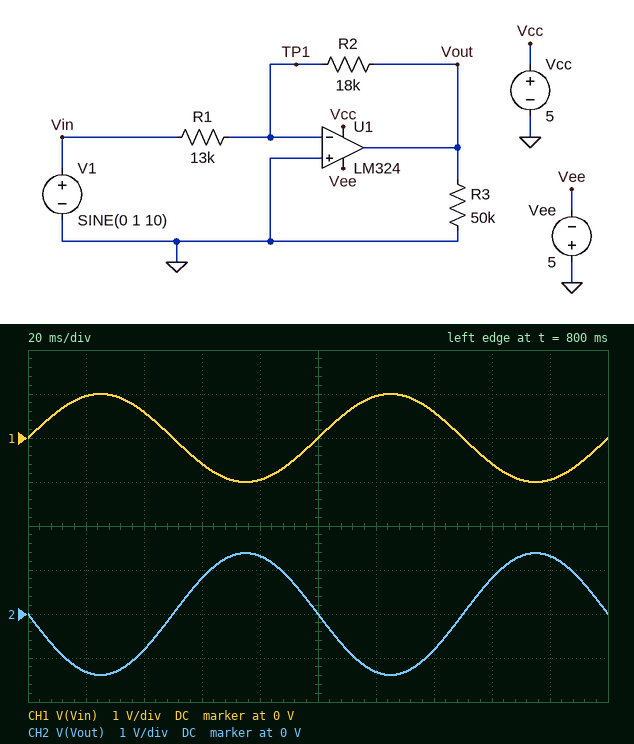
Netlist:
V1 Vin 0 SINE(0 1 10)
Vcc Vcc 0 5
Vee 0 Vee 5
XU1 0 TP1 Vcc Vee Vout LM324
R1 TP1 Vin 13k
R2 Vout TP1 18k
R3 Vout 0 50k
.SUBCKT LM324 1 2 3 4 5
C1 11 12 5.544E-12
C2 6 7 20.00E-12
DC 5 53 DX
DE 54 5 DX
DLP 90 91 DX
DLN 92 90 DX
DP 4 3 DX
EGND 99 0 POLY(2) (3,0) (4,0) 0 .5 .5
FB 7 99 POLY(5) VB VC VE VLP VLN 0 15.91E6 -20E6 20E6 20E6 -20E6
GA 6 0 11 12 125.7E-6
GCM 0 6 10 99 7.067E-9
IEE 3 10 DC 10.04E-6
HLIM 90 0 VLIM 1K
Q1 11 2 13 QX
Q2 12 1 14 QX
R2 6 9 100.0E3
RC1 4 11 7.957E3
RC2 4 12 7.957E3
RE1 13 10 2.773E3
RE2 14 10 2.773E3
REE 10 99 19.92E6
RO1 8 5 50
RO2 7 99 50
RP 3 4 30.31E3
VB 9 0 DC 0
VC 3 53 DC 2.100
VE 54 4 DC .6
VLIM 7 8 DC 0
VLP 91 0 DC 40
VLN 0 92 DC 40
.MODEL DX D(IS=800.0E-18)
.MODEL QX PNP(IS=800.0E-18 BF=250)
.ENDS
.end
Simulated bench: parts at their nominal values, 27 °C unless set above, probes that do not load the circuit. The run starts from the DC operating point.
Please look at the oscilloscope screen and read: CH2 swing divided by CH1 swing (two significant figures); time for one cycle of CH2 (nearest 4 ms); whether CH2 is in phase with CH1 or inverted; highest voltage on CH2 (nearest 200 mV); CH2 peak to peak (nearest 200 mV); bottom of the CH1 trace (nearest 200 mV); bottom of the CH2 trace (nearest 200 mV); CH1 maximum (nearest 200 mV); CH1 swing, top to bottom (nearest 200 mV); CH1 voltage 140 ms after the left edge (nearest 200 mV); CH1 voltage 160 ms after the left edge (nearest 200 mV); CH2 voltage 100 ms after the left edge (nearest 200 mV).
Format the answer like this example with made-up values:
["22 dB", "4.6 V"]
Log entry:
["1.4", "100 ms", "inverted", "1.4 V", "2.8 V", "-1.0 V", "-1.4 V", "1.0 V", "2.0 V", "600 mV", "-600 mV", "0 V"]
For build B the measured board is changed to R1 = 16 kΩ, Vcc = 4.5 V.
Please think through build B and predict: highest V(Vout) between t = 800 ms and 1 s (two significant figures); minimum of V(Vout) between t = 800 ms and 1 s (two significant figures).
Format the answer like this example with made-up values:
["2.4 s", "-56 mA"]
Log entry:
["1.1 V", "-1.1 V"]
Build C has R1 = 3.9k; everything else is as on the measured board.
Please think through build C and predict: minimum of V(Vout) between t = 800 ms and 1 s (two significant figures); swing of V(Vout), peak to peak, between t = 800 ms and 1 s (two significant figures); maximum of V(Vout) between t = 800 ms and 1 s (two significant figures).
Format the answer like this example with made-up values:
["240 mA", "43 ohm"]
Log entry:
["-4.6 V", "8.1 V", "3.5 V"]
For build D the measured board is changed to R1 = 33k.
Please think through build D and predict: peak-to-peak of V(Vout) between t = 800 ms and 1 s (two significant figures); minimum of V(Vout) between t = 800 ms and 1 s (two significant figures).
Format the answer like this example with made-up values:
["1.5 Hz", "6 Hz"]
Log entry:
["1.1 V", "-550 mV"]
